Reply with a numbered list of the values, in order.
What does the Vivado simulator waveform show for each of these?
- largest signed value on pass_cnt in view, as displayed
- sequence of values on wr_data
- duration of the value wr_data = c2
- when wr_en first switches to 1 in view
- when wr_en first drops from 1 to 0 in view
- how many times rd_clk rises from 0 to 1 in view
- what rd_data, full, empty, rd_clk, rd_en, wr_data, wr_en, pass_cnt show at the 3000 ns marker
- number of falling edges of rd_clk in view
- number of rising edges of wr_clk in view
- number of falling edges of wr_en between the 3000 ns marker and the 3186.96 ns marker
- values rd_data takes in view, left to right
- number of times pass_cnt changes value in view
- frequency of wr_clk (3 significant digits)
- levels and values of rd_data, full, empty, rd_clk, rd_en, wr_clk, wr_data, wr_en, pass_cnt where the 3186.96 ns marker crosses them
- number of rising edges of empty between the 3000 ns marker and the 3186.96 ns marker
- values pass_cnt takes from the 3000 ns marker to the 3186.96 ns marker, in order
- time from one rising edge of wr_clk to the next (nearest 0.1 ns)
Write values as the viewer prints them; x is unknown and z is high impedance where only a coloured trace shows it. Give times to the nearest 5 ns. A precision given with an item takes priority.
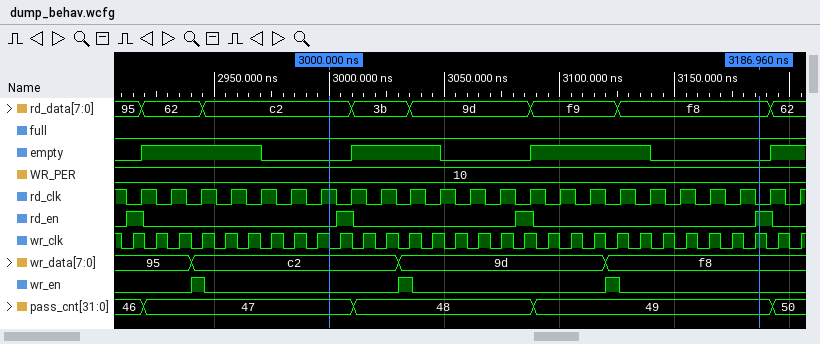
1. 50
2. 95, c2, 9d, f8
3. 90 ns
4. 2940 ns
5. 2945 ns
6. 23
7. rd_data=c2, full=0, empty=0, rd_clk=1, rd_en=0, wr_data=c2, wr_en=0, pass_cnt=47
8. 23
9. 30
10. 2
11. 95, 62, c2, 3b, 9d, f9, f8, 62
12. 4
13. 100 MHz
14. rd_data=f8, full=0, empty=0, rd_clk=0, rd_en=1, wr_clk=1, wr_data=f8, wr_en=0, pass_cnt=49
15. 2
16. 47, 48, 49
17. 10 ns
